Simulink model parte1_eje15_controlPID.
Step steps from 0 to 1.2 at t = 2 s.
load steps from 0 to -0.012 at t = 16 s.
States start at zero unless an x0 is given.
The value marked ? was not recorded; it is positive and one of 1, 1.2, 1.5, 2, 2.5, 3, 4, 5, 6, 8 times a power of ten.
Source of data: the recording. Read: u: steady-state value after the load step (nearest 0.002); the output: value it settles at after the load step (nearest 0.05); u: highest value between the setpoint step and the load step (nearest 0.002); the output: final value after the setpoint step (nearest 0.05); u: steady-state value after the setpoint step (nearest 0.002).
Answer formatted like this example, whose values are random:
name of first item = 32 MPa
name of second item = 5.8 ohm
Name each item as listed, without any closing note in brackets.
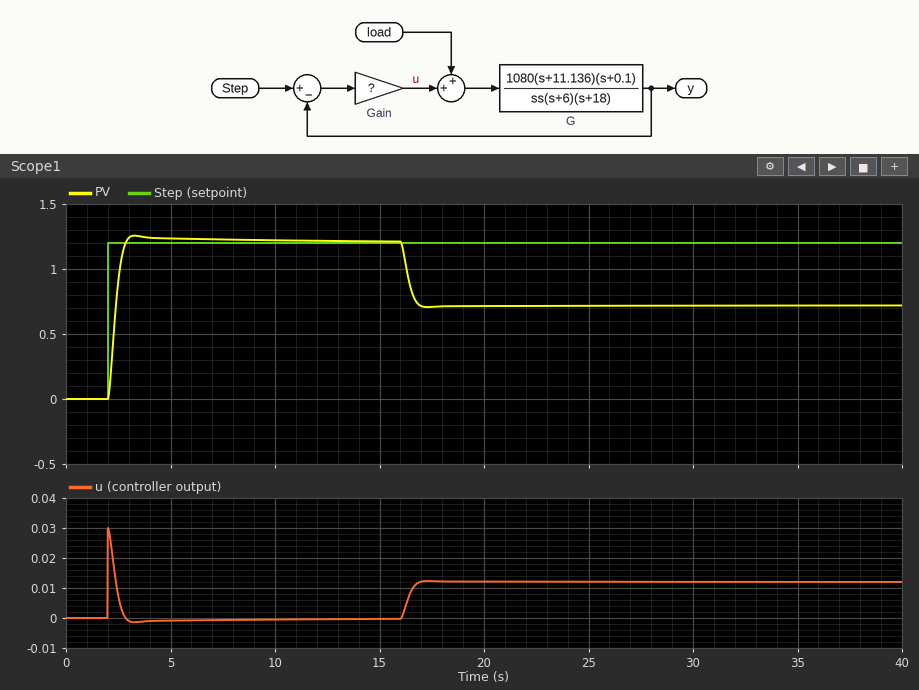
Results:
u: steady-state value after the load step = 0.012
the output: value it settles at after the load step = 0.70
u: highest value between the setpoint step and the load step = 0.030
the output: final value after the setpoint step = 1.20
u: steady-state value after the setpoint step = 0.000
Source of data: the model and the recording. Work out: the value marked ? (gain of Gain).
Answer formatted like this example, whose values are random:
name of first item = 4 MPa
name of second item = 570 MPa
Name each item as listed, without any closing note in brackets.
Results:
the value marked ? = 0.025
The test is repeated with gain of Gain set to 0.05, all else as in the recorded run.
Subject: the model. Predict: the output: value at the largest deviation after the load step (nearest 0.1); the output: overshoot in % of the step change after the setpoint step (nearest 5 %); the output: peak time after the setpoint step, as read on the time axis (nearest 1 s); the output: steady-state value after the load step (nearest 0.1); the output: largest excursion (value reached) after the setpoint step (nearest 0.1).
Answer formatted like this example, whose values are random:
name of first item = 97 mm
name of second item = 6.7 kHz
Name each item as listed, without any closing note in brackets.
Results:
the output: value at the largest deviation after the load step = 0.9
the output: overshoot in % of the step change after the setpoint step = 10 %
the output: peak time after the setpoint step, as read on the time axis = 3 s
the output: steady-state value after the load step = 1.0
the output: largest excursion (value reached) after the setpoint step = 1.3
